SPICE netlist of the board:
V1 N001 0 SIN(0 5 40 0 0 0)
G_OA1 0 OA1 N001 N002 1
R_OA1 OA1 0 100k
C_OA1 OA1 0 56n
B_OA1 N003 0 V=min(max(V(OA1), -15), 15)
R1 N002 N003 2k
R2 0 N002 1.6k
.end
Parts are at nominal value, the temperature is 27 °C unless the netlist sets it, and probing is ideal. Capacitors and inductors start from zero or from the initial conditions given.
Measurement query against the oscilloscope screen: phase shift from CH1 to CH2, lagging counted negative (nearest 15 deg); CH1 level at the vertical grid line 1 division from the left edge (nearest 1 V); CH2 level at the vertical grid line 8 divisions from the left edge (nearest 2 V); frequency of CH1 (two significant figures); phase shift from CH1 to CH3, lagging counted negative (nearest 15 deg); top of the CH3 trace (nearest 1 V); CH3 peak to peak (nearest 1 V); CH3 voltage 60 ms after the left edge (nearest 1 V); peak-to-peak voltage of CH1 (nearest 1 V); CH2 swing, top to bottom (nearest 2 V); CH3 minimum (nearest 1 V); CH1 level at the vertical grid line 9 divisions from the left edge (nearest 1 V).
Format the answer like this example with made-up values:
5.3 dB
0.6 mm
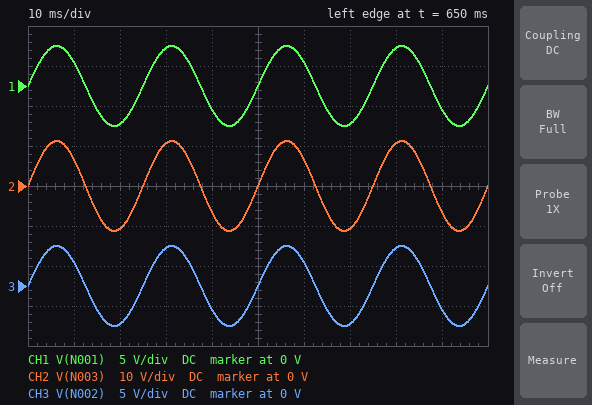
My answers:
0 deg
3 V
10 V
40 Hz
0 deg
5 V
10 V
3 V
10 V
22 V
-5 V
-3 V
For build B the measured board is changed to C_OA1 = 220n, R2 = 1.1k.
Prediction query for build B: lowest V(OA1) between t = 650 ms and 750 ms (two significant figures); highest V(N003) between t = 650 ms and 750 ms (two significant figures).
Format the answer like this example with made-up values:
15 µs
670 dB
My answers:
-14 V
14 V
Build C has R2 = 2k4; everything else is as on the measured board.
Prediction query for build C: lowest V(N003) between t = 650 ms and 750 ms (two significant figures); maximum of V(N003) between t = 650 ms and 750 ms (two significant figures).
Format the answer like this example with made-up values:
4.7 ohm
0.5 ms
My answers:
-9.2 V
9.2 V
